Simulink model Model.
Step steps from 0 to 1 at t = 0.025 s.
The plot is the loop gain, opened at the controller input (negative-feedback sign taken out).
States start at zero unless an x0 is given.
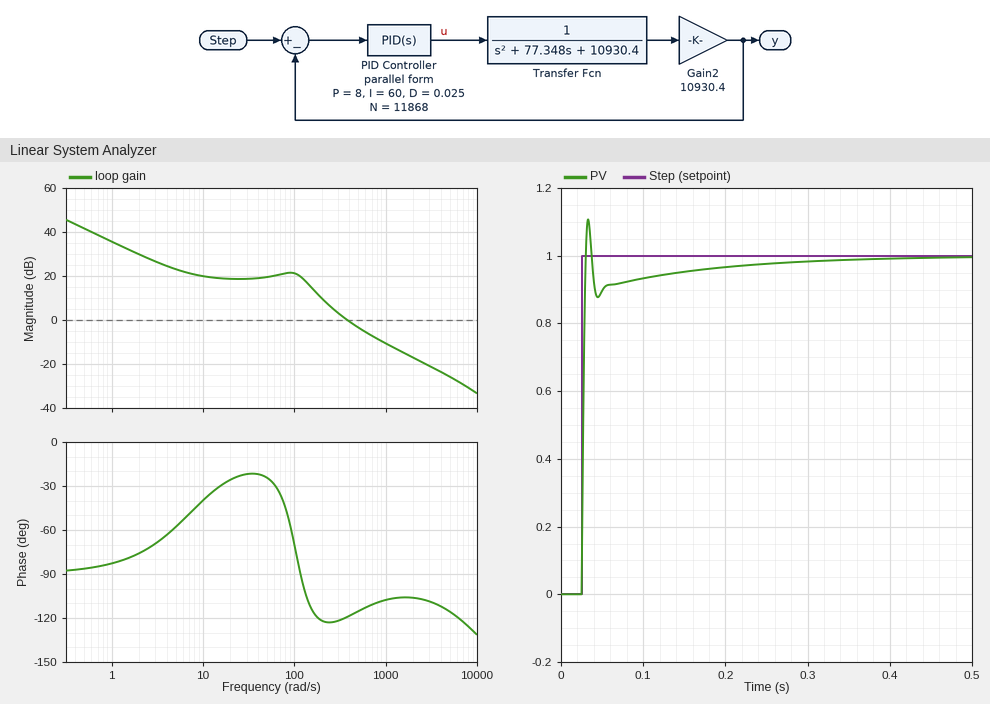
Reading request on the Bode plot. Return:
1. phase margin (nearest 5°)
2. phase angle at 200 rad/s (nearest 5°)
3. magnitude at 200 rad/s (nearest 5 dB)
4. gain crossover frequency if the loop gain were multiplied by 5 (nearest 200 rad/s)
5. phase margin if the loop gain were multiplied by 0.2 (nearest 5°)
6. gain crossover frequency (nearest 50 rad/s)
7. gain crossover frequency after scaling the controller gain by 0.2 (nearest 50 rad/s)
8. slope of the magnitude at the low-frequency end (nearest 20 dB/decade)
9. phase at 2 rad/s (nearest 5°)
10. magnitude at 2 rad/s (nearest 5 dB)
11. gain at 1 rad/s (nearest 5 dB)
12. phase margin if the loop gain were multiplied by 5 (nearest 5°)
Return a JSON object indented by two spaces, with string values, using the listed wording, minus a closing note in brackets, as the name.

{
  "phase margin": "60°",
  "phase angle at 200 rad/s": "-120°",
  "magnitude at 200 rad/s": "10 dB",
  "gain crossover frequency if the loop gain were multiplied by 5": "1400 rad/s",
  "phase margin if the loop gain were multiplied by 0.2": "65°",
  "gain crossover frequency": "400 rad/s",
  "gain crossover frequency after scaling the controller gain by 0.2": "150 rad/s",
  "slope of the magnitude at the low-frequency end": "-20 dB/decade",
  "phase at 2 rad/s": "-75°",
  "magnitude at 2 rad/s": "30 dB",
  "gain at 1 rad/s": "35 dB",
  "phase margin if the loop gain were multiplied by 5": "75°"
}
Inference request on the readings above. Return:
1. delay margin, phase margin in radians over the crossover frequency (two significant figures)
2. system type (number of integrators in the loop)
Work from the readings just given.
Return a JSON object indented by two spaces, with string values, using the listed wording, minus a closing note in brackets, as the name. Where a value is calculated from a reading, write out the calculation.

{
  "delay margin, phase margin in radians over the crossover frequency": "60 × π / 180 / 400 = 0.0026 s",
  "system type": "1"
}
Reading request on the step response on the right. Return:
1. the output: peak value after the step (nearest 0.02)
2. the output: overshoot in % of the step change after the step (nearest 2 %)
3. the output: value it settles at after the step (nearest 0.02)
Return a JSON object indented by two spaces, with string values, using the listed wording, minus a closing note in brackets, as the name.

{
  "the output: peak value after the step": "1.10",
  "the output: overshoot in % of the step change after the step": "10 %",
  "the output: value it settles at after the step": "1.00"
}
